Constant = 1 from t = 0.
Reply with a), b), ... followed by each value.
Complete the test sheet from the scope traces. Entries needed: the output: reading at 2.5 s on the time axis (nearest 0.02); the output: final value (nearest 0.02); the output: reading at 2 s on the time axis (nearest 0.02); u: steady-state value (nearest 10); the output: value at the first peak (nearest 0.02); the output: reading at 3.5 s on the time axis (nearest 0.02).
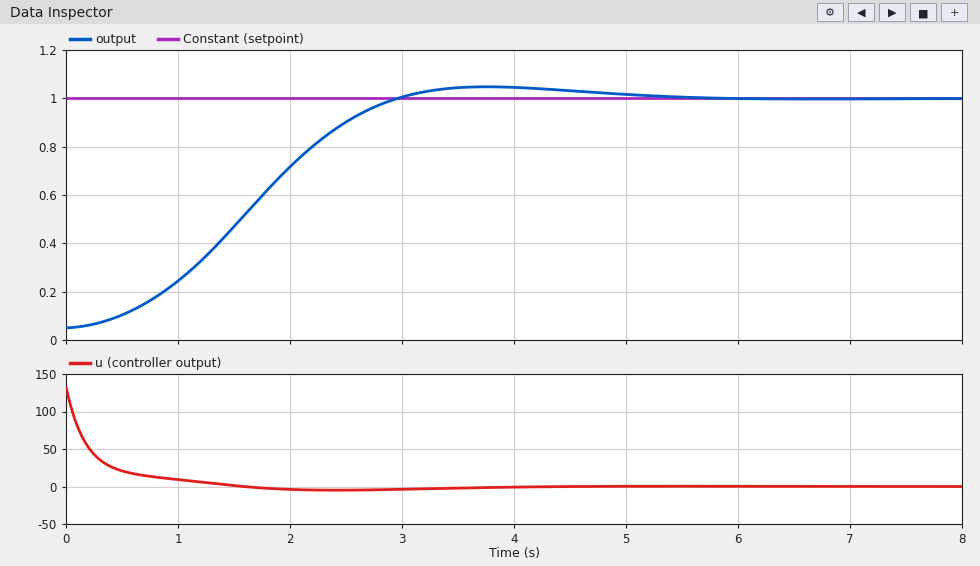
a) 0.90
b) 1.00
c) 0.72
d) 0
e) 1.04
f) 1.04
